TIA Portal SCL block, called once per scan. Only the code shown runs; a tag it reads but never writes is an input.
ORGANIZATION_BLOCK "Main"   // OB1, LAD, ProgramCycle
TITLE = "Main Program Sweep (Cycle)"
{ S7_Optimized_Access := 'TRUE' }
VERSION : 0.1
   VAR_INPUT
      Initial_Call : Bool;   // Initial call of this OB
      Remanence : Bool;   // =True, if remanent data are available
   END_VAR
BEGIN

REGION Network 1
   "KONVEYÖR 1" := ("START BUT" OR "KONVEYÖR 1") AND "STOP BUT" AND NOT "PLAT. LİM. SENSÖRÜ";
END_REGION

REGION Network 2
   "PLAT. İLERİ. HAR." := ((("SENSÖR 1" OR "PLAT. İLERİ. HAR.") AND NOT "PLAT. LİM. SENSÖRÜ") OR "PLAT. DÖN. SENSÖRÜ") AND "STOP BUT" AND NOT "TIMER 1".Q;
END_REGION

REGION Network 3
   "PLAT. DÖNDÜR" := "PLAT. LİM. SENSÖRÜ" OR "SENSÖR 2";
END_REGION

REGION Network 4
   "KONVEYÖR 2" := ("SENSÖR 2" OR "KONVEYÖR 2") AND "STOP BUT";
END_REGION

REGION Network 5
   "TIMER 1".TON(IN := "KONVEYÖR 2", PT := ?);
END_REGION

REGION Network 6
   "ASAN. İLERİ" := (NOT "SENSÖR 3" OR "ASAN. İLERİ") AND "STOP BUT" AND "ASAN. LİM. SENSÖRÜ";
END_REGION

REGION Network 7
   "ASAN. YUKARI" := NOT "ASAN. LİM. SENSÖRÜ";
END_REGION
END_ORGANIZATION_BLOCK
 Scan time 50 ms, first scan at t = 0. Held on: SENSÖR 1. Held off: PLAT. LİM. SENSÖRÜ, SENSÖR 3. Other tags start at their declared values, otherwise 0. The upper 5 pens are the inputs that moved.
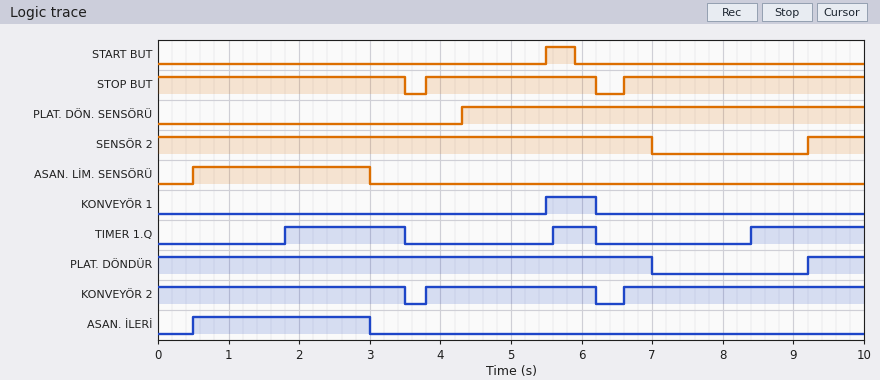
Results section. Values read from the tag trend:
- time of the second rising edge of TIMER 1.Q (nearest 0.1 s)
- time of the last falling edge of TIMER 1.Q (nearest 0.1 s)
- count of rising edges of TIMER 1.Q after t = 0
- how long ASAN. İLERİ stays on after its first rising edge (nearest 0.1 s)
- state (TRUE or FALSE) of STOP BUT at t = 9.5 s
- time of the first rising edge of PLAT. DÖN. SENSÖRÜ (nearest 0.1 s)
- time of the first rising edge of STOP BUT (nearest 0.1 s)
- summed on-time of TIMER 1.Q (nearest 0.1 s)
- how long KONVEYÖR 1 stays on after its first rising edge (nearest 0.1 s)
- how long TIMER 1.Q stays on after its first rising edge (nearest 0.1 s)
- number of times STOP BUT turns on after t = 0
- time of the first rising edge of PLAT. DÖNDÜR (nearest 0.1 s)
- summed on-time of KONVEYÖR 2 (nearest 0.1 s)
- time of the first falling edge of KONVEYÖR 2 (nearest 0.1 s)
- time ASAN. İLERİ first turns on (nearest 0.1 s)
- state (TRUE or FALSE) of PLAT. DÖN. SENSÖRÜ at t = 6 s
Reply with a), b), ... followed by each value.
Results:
a) 5.6 s
b) 6.2 s
c) 3
d) 2.5 s
e) TRUE
f) 4.3 s
g) 3.8 s
h) 3.9 s
i) 0.7 s
j) 1.7 s
k) 2
l) 9.2 s
m) 9.3 s
n) 3.5 s
o) 0.5 s
p) TRUE
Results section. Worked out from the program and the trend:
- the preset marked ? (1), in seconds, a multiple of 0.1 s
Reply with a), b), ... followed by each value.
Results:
a) 1.8 s
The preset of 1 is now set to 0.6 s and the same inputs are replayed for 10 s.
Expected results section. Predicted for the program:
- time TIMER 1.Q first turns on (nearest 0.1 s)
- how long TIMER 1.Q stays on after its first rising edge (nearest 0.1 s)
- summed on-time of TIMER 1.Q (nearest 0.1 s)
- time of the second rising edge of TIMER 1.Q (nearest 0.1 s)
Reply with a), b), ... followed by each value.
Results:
a) 0.6 s
b) 2.9 s
c) 7.5 s
d) 4.4 s
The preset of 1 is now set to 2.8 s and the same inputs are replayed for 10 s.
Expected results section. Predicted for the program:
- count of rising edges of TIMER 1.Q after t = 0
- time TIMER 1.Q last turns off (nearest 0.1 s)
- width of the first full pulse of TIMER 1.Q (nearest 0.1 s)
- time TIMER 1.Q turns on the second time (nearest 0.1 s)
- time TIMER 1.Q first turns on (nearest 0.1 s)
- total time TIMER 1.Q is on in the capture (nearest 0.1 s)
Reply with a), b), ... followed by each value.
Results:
a) 2
b) 3.5 s
c) 0.7 s
d) 9.4 s
e) 2.8 s
f) 1.3 s
